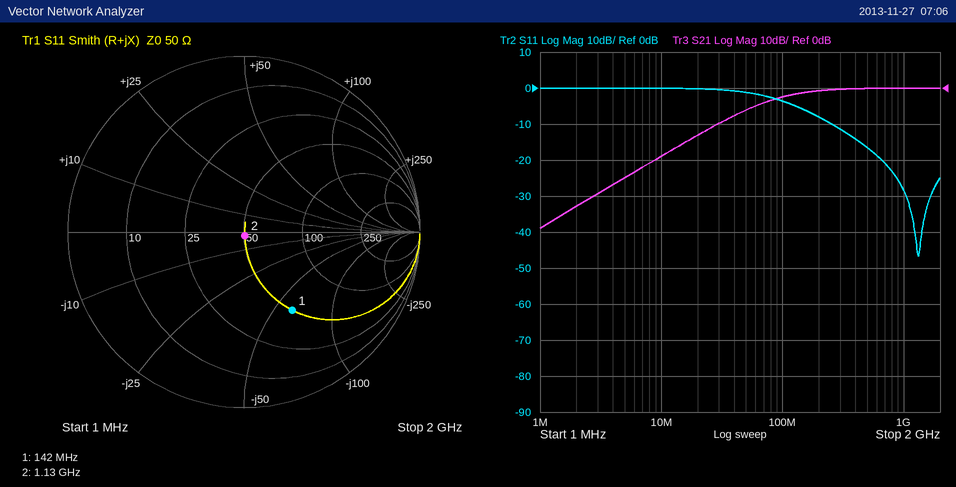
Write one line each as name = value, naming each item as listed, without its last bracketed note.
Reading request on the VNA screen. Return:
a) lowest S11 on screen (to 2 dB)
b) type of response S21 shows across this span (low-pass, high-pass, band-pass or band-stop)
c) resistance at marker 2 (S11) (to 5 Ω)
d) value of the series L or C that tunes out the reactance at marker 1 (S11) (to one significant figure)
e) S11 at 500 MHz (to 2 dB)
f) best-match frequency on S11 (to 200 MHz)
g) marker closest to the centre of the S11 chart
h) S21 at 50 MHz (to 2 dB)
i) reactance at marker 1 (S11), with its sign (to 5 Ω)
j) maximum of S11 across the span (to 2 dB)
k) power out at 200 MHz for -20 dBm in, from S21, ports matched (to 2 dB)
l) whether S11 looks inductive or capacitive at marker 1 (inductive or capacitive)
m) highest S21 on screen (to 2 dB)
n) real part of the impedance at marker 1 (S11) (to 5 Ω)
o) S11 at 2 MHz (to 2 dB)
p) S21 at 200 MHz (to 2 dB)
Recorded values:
lowest S11 on screen = -46 dB
type of response S21 shows across this span = high-pass
resistance at marker 2 (S11) = 50 Ω
value of the series L or C that tunes out the reactance at marker 1 (S11) = 70 nH
S11 at 500 MHz = -16 dB
best-match frequency on S11 = 1.4 GHz
marker closest to the centre of the S11 chart = marker 2
S21 at 50 MHz = -6 dB
reactance at marker 1 (S11), with its sign = -60 Ω
maximum of S11 across the span = 0 dB
power out at 200 MHz for -20 dBm in, from S21, ports matched = -20 dBm
whether S11 looks inductive or capacitive at marker 1 = capacitive
highest S21 on screen = 0 dB
real part of the impedance at marker 1 (S11) = 50 Ω
S11 at 2 MHz = 0 dB
S21 at 200 MHz = 0 dB
